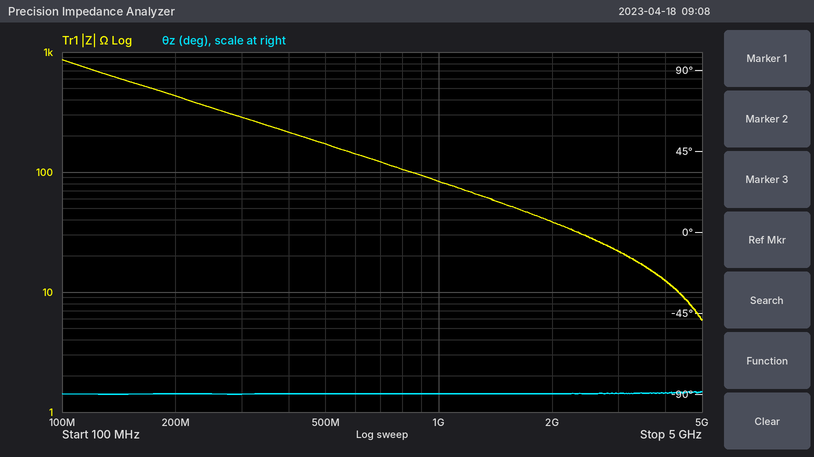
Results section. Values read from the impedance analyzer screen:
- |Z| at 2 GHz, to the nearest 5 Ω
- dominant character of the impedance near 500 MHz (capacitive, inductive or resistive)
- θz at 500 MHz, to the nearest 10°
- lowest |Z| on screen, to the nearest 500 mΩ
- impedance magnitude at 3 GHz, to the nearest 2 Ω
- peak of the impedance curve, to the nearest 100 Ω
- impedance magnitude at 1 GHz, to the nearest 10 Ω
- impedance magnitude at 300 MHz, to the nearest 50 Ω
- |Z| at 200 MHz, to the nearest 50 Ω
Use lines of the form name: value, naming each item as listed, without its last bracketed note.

|Z| at 2 GHz, to the nearest 5 Ω: 40 Ω
dominant character of the impedance near 500 MHz: capacitive
θz at 500 MHz, to the nearest 10°: -90°
lowest |Z| on screen, to the nearest 500 mΩ: 6.0 Ω
impedance magnitude at 3 GHz, to the nearest 2 Ω: 22 Ω
peak of the impedance curve, to the nearest 100 Ω: 900 Ω
impedance magnitude at 1 GHz, to the nearest 10 Ω: 80 Ω
impedance magnitude at 300 MHz, to the nearest 50 Ω: 300 Ω
|Z| at 200 MHz, to the nearest 50 Ω: 450 Ω
